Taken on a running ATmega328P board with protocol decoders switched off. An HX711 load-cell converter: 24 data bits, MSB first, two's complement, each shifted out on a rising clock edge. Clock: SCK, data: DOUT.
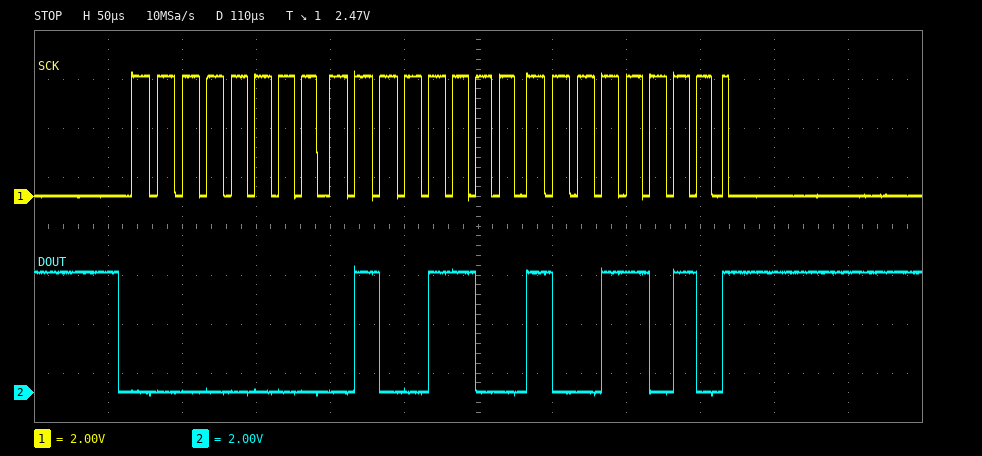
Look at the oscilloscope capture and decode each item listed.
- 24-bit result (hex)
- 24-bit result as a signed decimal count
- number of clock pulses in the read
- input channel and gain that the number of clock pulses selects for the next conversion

0x004C9A
19610
25
channel A, gain 128
